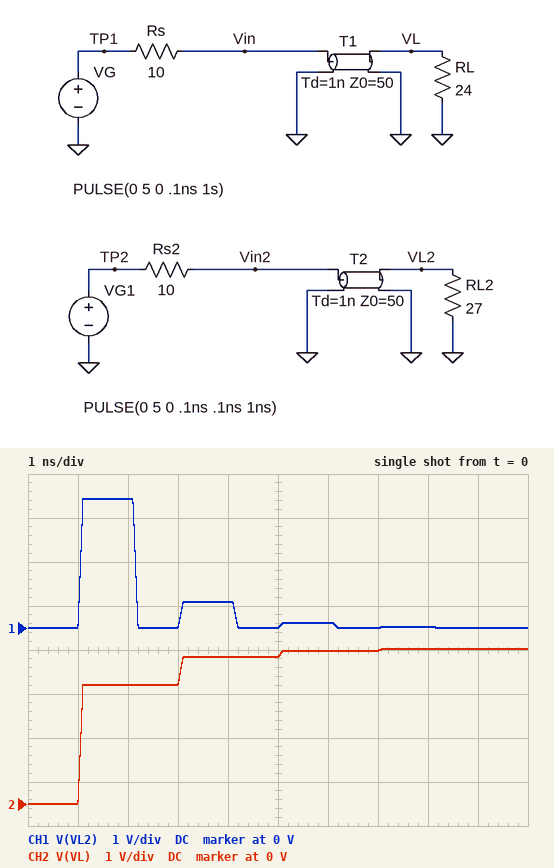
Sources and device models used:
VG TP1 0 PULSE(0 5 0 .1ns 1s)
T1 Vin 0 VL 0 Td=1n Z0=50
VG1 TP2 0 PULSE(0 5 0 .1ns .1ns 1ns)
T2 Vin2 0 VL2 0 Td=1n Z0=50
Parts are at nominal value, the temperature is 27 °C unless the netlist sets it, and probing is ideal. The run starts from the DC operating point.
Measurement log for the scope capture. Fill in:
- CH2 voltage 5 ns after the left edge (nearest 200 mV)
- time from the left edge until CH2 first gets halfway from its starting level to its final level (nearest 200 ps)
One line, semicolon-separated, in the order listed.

3.4 V; 1.0 ns
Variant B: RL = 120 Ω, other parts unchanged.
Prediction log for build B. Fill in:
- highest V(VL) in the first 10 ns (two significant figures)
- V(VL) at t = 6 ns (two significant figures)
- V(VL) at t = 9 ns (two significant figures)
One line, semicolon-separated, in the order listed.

5.9 V; 4.7 V; 4.6 V
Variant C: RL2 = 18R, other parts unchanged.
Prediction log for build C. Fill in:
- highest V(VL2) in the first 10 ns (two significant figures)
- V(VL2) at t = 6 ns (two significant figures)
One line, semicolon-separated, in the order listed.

2.2 V; 220 mV
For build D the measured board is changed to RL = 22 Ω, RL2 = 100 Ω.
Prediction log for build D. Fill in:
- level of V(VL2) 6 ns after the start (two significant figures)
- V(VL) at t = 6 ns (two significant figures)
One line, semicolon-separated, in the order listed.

270 mV; 3.4 V
